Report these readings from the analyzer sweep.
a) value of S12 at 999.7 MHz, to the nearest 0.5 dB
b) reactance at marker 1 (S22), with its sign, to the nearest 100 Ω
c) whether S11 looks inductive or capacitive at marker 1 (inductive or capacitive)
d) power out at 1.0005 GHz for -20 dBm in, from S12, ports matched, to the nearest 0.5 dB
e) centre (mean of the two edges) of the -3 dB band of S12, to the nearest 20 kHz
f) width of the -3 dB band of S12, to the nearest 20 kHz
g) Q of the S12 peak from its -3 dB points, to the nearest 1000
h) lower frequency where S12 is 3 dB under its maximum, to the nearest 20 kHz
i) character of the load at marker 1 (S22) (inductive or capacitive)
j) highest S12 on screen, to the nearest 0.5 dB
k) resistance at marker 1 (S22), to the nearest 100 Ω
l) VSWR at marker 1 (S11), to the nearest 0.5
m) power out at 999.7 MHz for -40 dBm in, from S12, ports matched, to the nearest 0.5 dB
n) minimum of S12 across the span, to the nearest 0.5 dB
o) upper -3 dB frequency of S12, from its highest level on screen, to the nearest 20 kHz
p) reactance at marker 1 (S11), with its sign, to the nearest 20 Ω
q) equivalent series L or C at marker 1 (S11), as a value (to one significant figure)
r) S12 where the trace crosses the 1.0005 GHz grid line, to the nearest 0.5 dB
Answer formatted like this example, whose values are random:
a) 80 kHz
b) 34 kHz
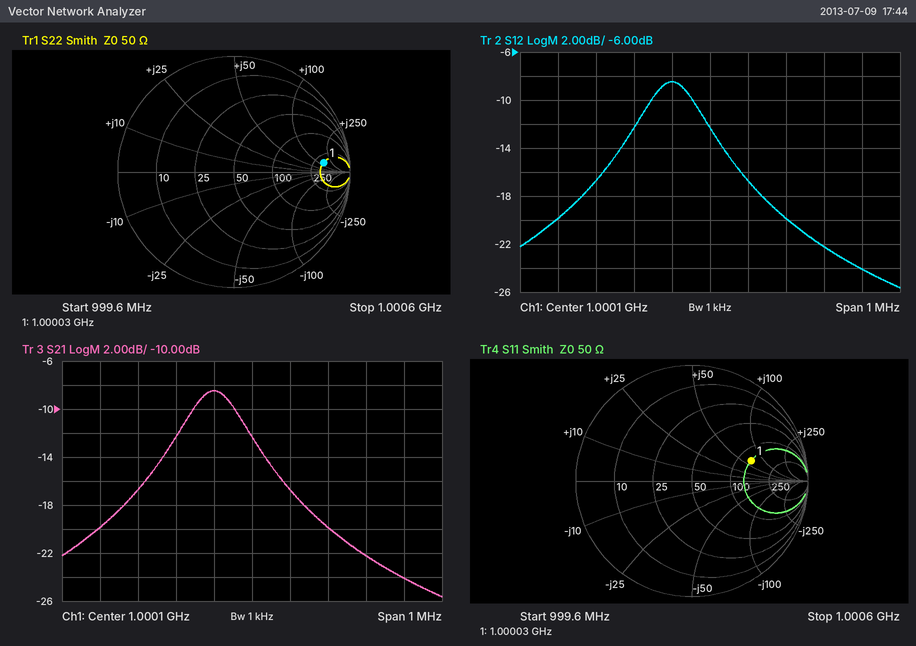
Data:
a) -20.0 dB
b) +100 Ω
c) inductive
d) -44.0 dBm
e) 1.00000 GHz
f) 160 kHz
g) 6000
h) 999.92 MHz
i) inductive
j) -8.5 dB
k) 300 Ω
l) 3.5
m) -60.0 dBm
n) -25.5 dB
o) 1.00008 GHz
p) +60 Ω
q) 10 nH
r) -24.0 dB
